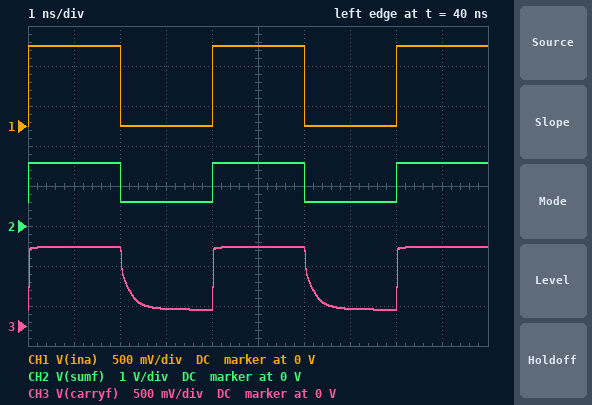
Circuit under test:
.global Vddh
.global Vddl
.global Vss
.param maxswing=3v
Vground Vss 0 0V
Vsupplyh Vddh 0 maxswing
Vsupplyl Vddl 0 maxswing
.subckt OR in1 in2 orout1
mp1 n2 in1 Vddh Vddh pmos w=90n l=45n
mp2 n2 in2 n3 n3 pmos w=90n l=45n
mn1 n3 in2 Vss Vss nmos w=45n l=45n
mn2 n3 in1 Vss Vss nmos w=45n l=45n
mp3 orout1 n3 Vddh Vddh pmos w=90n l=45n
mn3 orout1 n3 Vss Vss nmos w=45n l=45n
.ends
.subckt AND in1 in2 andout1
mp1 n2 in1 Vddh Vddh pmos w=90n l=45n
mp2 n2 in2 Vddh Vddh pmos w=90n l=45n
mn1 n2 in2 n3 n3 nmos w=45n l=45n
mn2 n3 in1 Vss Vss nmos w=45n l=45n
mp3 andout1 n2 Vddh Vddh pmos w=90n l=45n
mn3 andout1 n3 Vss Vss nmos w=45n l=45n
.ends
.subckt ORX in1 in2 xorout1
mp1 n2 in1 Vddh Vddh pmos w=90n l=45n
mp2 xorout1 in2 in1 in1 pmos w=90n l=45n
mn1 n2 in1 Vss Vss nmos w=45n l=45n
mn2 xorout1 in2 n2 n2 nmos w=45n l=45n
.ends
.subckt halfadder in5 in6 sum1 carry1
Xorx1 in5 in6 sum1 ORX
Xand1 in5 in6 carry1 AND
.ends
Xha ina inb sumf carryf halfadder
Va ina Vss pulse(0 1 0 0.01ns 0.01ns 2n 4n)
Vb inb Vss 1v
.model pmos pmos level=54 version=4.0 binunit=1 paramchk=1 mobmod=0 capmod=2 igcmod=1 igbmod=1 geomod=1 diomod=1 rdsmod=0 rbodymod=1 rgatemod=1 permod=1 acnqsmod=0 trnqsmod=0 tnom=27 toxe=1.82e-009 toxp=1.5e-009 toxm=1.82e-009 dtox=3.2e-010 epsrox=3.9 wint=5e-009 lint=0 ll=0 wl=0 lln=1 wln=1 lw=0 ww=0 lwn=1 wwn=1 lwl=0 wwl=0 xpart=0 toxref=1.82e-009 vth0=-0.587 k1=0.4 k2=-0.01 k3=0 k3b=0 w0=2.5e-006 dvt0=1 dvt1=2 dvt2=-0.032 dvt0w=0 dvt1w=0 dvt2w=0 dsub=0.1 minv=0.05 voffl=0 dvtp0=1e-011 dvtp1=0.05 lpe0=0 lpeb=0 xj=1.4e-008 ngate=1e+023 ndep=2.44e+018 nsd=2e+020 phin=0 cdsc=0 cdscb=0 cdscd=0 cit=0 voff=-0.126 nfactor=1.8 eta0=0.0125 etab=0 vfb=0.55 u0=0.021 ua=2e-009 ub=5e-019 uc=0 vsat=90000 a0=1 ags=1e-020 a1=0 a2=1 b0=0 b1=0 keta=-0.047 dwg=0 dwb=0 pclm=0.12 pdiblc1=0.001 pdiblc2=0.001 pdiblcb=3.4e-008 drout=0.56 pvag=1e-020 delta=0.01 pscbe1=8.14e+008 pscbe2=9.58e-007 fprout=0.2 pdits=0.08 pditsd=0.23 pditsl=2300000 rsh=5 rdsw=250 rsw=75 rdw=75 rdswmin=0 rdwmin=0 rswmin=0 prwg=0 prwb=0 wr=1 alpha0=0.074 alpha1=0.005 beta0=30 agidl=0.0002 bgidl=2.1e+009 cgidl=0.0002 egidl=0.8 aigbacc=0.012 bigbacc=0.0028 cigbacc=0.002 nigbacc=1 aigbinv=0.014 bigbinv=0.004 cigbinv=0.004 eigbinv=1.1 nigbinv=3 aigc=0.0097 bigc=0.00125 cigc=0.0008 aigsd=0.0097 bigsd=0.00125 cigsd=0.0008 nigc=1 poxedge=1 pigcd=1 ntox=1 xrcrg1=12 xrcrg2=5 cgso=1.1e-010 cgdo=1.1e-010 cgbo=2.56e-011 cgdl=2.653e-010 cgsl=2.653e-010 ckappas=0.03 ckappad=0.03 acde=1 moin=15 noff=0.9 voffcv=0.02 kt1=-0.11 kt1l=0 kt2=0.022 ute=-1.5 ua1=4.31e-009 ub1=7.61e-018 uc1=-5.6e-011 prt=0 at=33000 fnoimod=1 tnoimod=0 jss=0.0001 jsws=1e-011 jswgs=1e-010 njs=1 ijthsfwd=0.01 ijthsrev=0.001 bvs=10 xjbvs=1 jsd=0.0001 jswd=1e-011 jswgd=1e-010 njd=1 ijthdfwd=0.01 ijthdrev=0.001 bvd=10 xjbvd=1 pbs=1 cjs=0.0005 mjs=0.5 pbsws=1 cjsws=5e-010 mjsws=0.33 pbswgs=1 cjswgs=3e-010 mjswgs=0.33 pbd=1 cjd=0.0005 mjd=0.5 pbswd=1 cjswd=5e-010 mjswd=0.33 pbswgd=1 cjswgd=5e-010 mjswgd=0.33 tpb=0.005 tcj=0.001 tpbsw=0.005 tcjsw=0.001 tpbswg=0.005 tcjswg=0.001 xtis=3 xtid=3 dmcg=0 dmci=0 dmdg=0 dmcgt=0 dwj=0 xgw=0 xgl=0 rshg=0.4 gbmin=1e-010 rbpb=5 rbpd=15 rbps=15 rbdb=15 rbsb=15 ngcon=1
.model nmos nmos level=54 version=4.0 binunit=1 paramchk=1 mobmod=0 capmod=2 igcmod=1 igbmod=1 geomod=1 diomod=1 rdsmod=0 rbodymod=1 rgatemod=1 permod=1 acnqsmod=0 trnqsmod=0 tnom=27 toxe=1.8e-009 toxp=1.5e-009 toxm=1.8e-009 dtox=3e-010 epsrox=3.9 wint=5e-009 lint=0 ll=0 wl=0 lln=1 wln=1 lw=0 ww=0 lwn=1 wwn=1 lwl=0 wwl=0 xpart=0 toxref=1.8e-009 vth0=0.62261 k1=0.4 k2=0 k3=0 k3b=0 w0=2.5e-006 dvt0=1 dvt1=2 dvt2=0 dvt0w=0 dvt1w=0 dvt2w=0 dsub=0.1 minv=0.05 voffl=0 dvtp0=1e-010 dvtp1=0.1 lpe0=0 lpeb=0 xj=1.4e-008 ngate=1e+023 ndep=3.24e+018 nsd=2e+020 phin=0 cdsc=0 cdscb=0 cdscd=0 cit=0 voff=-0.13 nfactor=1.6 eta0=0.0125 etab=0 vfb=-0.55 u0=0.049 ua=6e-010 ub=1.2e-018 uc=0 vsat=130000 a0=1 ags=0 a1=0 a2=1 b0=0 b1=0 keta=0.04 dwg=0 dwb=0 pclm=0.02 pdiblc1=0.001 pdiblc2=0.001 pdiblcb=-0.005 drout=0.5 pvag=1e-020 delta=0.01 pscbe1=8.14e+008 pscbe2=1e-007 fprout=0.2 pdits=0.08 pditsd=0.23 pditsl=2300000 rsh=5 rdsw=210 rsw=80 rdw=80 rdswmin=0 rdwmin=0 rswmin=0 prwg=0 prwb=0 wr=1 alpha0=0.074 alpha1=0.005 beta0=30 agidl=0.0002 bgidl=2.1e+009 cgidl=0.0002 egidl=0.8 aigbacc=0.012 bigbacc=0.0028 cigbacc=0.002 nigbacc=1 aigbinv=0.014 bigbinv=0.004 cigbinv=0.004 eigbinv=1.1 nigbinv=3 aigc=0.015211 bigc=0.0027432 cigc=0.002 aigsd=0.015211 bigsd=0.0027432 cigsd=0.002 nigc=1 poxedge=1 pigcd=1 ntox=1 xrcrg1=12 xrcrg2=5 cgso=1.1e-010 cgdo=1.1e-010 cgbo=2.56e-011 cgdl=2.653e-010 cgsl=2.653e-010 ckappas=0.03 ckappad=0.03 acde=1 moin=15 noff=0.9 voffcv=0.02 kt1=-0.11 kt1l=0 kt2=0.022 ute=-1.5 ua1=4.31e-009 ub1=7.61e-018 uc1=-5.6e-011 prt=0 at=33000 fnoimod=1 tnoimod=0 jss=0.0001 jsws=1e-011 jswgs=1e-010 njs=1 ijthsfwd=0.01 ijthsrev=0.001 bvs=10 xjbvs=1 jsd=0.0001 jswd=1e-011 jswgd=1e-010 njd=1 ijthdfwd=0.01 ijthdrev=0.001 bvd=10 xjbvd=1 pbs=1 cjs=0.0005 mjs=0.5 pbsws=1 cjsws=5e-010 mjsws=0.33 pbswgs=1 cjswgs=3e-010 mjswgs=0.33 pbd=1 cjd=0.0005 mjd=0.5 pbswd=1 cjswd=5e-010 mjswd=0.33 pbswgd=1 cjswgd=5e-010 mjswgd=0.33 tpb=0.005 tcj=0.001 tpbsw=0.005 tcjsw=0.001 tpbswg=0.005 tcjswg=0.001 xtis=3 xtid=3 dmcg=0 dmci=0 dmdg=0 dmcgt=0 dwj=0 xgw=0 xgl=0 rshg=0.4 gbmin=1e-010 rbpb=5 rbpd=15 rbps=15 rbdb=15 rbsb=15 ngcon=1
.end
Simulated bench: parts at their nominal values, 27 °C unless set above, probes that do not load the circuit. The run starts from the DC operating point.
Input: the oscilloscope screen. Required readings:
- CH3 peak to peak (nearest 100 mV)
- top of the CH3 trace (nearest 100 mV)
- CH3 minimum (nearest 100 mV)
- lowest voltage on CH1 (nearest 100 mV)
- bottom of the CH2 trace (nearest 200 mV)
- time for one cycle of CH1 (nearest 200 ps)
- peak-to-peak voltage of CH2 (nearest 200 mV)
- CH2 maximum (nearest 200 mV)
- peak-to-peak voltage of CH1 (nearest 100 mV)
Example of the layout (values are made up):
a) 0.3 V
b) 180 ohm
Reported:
a) 800 mV
b) 1.0 V
c) 200 mV
d) 0 V
e) 600 mV
f) 4.0 ns
g) 1.0 V
h) 1.6 V
i) 1.0 V
